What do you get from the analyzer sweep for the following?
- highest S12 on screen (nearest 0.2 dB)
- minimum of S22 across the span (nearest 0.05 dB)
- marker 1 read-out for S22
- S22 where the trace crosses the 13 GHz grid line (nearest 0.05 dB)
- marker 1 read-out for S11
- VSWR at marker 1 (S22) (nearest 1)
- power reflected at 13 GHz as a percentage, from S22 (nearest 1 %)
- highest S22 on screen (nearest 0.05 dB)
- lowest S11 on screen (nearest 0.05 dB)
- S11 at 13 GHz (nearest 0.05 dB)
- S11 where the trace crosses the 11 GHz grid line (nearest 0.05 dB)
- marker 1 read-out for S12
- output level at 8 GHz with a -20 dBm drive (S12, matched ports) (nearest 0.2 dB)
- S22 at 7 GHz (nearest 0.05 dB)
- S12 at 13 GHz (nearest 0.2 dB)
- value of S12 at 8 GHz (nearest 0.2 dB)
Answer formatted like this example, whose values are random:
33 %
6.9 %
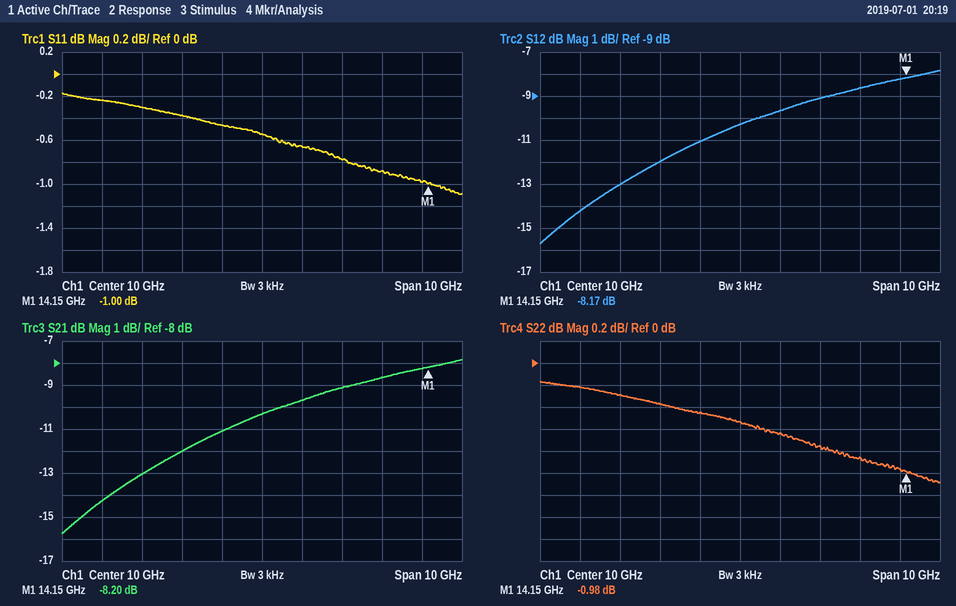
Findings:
-7.8 dB
-1.10 dB
-0.98 dB
-0.85 dB
-1.00 dB
18
82 %
-0.15 dB
-1.10 dB
-0.90 dB
-0.65 dB
-8.17 dB
-32.0 dBm
-0.30 dB
-8.6 dB
-12.0 dB
